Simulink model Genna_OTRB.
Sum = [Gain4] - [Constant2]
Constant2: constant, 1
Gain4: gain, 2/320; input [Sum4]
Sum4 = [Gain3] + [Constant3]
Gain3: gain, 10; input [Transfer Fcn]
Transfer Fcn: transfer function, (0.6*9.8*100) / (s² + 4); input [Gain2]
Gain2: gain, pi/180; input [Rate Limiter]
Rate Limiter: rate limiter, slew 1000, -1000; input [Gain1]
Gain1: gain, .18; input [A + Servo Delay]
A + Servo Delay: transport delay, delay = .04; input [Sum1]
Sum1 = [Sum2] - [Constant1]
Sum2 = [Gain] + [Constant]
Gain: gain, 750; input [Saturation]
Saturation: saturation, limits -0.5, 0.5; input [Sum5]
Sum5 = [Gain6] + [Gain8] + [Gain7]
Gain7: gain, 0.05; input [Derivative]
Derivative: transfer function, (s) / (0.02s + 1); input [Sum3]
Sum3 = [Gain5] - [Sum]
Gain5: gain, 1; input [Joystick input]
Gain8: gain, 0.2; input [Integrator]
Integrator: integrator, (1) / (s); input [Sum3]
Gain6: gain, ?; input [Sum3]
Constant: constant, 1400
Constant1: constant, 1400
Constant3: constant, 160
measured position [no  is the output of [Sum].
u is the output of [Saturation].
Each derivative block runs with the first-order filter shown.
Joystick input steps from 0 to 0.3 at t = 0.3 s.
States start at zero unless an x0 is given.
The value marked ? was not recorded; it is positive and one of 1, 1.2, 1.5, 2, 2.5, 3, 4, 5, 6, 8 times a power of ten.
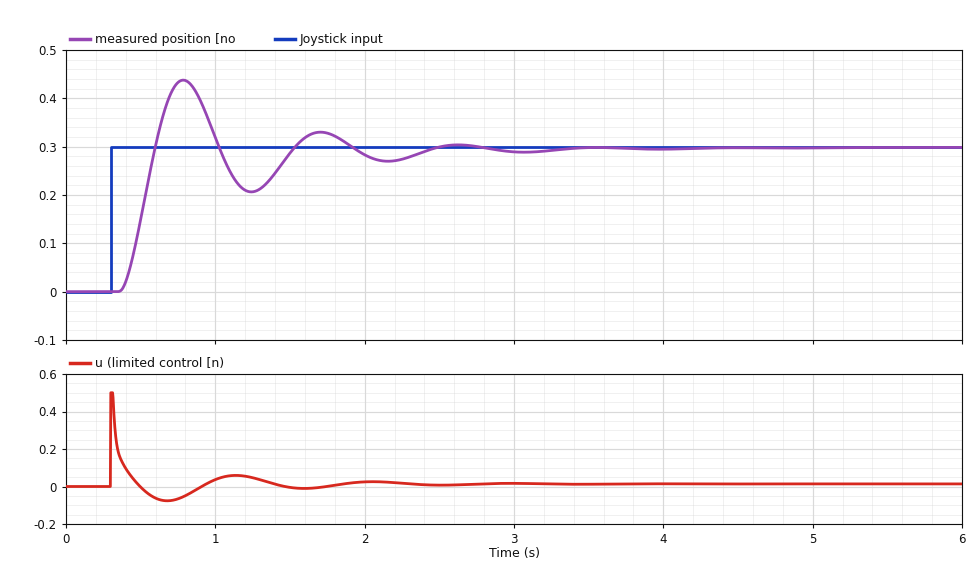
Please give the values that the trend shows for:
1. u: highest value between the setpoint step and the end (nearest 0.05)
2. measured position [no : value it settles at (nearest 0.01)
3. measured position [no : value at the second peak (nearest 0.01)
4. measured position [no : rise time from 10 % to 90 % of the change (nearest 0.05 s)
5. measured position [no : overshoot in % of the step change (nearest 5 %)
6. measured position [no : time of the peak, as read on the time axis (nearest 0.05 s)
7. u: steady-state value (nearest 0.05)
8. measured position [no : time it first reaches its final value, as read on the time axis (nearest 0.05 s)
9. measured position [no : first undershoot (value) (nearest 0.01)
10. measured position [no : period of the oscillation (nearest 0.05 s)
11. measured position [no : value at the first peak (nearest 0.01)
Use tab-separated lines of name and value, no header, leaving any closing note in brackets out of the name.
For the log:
u: highest value between the setpoint step and the end	0.50
measured position [no : value it settles at	0.30
measured position [no : value at the second peak	0.33
measured position [no : rise time from 10 % to 90 % of the change	0.15 s
measured position [no : overshoot in % of the step change	45 %
measured position [no : time of the peak, as read on the time axis	0.80 s
u: steady-state value	0.00
measured position [no : time it first reaches its final value, as read on the time axis	0.60 s
measured position [no : first undershoot (value)	0.21
measured position [no : period of the oscillation	0.90 s
measured position [no : value at the first peak	0.44
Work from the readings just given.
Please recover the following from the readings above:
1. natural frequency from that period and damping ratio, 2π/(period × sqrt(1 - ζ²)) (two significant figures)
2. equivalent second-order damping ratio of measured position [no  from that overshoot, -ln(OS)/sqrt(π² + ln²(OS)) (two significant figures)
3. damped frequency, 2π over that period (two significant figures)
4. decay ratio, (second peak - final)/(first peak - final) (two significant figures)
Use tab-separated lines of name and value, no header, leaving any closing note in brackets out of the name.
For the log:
natural frequency from that period and damping ratio, 2π/(period × sqrt(1 - ζ²))	7.2 rad/s
equivalent second-order damping ratio of measured position [no  from that overshoot, -ln(OS)/sqrt(π² + ln²(OS))	0.25
damped frequency, 2π over that period	7.0 rad/s
decay ratio, (second peak - final)/(first peak - final)	0.21
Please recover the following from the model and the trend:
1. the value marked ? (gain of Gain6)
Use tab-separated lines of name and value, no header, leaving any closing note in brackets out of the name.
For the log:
the value marked ?	0.4
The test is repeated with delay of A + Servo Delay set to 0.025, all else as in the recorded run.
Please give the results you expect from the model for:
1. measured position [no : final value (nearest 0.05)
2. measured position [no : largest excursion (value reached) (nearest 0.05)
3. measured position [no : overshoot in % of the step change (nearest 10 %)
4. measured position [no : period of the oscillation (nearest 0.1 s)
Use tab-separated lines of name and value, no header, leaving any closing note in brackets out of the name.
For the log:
measured position [no : final value	0.30
measured position [no : largest excursion (value reached)	0.40
measured position [no : overshoot in % of the step change	40 %
measured position [no : period of the oscillation	1.0 s
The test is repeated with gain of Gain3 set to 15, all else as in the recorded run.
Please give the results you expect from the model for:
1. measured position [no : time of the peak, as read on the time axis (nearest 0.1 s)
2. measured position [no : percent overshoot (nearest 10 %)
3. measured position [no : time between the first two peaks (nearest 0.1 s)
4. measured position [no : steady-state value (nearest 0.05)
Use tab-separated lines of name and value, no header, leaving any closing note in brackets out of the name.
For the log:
measured position [no : time of the peak, as read on the time axis	0.7 s
measured position [no : percent overshoot	40 %
measured position [no : time between the first two peaks	0.7 s
measured position [no : steady-state value	0.30
